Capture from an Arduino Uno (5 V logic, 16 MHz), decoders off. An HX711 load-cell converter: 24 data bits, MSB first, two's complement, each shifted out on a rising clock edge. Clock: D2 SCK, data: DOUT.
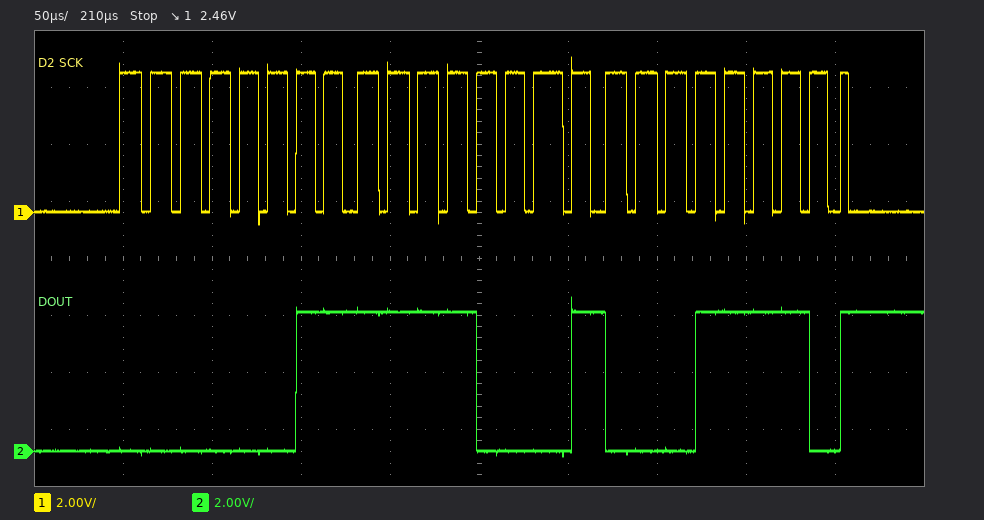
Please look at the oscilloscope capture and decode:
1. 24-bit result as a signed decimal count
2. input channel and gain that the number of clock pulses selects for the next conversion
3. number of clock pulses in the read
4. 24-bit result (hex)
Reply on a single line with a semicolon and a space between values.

258334; channel A, gain 128; 25; 0x03F11E
